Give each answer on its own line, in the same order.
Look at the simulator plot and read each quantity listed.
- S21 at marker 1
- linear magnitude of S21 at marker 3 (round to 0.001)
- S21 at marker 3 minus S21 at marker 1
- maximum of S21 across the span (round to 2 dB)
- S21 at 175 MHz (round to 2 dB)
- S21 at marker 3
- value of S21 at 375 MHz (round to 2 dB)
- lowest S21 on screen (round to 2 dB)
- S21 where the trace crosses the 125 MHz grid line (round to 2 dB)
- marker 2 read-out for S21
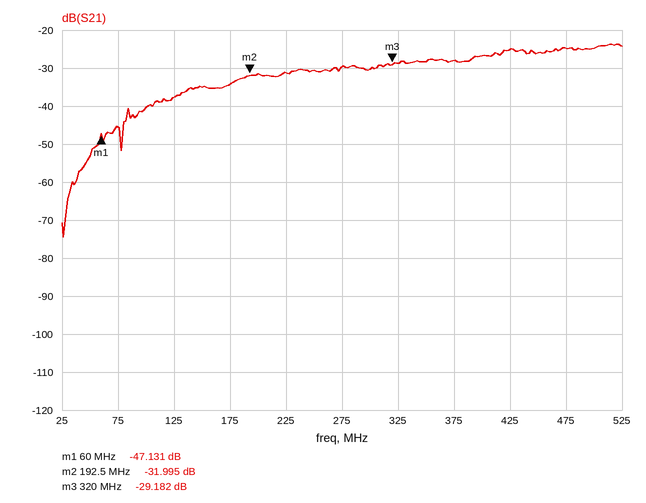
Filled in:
-47.131 dB
0.035
17.949 dB
-24 dB
-34 dB
-29.182 dB
-28 dB
-74 dB
-38 dB
-31.995 dB
